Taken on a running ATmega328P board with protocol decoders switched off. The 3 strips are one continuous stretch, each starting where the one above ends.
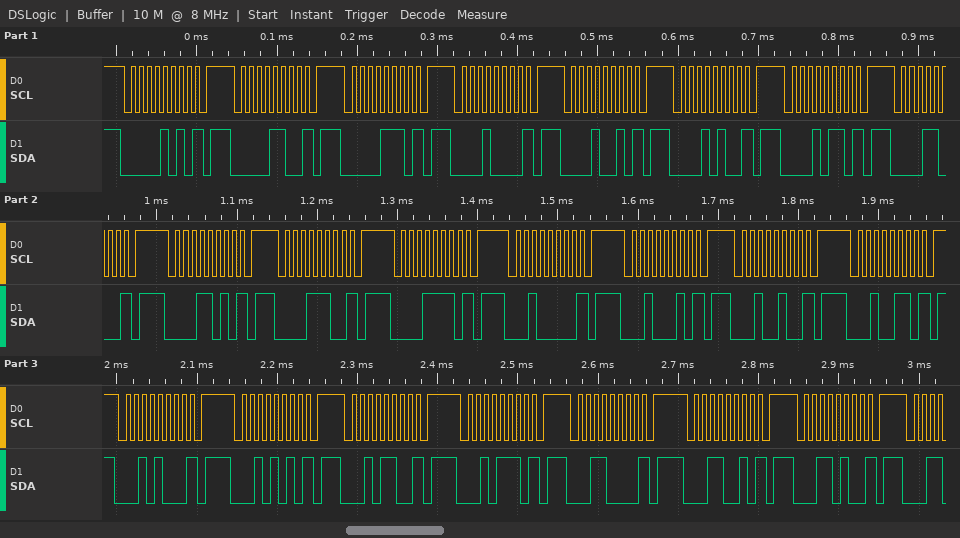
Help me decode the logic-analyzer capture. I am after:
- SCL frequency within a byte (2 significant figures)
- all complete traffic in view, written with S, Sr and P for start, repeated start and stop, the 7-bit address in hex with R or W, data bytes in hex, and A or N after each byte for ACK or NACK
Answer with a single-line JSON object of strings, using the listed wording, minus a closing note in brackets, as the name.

{"SCL frequency within a byte": "100 kHz", "all complete traffic in view, written with S, Sr and P for start, repeated start and stop, the 7-bit address in hex with R or W, data bytes in hex, and A or N after each byte for ACK or NACK": "S 05W N P S 06W N P S 07W N P S 08W N P S 09W N P S 0AW N P S 0BW N P S 0CW N P S 0DW N P S 0EW N P S 0FW N P S 10W N P S 11W N P S 12W N P S 13W N P S 14W N P S 15W N P S 16W N P S 17W N P S 18W N P S 19W N P S 1AW N P"}
